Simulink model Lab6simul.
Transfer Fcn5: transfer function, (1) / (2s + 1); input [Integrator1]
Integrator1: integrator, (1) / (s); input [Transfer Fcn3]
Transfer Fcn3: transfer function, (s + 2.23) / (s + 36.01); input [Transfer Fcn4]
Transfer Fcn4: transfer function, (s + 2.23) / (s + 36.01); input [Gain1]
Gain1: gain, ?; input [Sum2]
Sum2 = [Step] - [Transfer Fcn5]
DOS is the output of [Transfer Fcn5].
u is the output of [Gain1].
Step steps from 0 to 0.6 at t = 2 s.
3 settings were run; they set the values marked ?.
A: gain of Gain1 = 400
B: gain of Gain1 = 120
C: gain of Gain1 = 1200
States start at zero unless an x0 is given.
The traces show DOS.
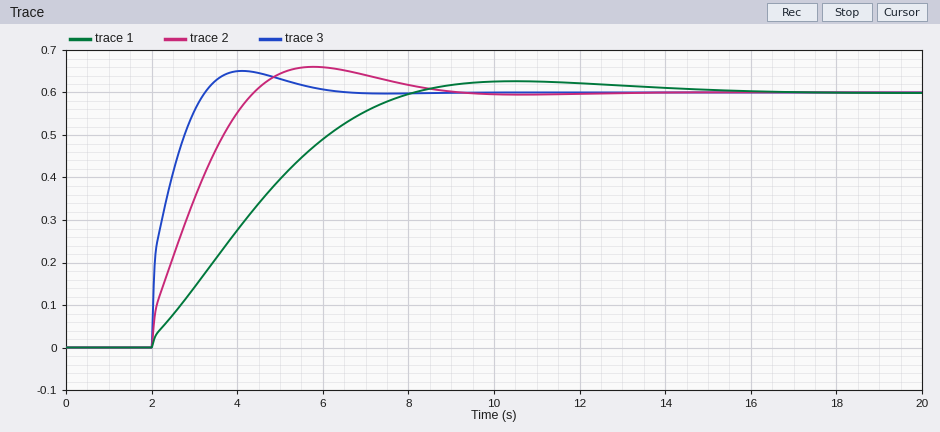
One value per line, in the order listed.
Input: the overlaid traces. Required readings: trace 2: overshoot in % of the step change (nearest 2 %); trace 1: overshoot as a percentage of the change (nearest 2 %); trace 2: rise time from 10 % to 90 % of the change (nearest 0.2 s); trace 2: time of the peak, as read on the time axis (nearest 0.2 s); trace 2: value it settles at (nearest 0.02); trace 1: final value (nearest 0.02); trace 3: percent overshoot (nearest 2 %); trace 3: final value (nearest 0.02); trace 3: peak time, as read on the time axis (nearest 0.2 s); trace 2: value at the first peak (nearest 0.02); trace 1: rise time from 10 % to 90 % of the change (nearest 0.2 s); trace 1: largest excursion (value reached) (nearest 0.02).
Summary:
10 %
4 %
1.8 s
5.8 s
0.60
0.60
8 %
0.60
4.2 s
0.66
4.4 s
0.62
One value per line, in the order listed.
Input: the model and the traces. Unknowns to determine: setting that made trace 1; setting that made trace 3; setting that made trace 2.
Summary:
B
C
A
